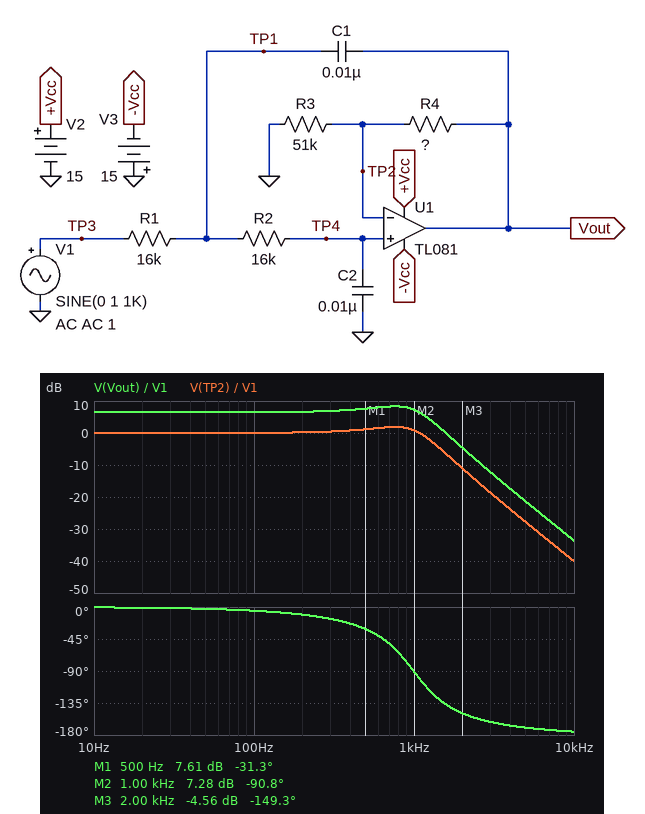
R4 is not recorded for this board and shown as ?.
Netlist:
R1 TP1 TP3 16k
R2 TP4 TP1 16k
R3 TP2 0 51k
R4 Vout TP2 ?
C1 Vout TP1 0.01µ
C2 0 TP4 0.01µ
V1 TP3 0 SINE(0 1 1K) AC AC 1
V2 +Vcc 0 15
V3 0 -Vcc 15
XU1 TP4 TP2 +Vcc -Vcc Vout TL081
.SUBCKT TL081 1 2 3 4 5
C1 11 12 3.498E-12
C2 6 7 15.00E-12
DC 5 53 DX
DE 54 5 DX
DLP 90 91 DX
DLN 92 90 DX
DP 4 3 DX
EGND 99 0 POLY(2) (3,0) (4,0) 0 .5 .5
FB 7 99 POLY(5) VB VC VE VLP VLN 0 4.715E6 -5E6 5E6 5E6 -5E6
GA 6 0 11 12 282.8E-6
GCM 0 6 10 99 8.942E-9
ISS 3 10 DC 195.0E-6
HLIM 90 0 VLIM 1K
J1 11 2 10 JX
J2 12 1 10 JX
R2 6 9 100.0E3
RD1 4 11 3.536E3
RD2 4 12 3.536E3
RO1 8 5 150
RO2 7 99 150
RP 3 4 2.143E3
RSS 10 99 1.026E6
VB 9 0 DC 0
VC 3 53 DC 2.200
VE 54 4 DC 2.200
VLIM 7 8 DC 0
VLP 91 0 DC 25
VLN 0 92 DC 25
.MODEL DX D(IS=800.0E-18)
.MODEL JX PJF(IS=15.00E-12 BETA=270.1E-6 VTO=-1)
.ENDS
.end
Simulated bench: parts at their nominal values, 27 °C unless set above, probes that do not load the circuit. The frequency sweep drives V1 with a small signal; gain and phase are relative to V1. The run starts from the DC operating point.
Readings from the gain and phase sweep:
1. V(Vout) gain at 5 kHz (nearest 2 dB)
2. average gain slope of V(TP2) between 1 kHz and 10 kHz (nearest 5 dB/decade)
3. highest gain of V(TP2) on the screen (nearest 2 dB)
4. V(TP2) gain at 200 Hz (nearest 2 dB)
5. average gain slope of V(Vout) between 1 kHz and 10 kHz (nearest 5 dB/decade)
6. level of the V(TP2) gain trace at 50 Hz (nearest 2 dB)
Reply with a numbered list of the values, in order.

1. -22 dB
2. -40 dB/decade
3. 2 dB
4. 0 dB
5. -40 dB/decade
6. 0 dB
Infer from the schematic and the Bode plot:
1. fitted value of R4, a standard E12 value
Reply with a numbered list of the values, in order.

1. 56 kΩ
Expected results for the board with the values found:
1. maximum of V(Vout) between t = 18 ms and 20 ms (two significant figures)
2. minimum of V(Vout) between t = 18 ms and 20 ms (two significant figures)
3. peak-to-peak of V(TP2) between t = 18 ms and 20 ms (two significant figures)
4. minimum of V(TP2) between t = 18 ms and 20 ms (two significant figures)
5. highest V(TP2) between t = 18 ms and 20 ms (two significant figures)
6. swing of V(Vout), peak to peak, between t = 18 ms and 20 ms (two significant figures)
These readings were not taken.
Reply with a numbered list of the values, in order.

1. 2.3 V
2. -2.3 V
3. 2.2 V
4. -1.1 V
5. 1.1 V
6. 4.6 V
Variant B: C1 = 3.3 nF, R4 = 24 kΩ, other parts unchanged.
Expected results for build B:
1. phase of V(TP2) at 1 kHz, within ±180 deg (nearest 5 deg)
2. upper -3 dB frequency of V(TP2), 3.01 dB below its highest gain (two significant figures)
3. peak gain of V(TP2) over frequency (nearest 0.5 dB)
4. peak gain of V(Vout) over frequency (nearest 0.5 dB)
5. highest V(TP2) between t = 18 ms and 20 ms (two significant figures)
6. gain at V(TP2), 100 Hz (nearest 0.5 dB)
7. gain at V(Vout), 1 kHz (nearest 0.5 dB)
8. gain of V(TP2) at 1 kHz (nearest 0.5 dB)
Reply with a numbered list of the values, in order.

1. -70 deg
2. 600 Hz
3. 0 dB
4. 3.5 dB
5. 510 mV
6. 0 dB
7. -2.5 dB
8. -6.0 dB
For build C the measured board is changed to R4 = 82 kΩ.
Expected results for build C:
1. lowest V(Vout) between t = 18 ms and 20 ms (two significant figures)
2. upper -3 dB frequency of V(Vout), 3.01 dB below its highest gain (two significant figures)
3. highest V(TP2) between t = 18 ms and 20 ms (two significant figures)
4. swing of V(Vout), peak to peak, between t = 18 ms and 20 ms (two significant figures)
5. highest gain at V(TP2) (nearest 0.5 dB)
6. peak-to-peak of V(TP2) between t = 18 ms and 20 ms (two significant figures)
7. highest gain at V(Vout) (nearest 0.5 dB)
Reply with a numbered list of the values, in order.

1. -6.6 V
2. 1.1 kHz
3. 2.5 V
4. 13 V
5. 8.5 dB
6. 5.1 V
7. 16.5 dB
